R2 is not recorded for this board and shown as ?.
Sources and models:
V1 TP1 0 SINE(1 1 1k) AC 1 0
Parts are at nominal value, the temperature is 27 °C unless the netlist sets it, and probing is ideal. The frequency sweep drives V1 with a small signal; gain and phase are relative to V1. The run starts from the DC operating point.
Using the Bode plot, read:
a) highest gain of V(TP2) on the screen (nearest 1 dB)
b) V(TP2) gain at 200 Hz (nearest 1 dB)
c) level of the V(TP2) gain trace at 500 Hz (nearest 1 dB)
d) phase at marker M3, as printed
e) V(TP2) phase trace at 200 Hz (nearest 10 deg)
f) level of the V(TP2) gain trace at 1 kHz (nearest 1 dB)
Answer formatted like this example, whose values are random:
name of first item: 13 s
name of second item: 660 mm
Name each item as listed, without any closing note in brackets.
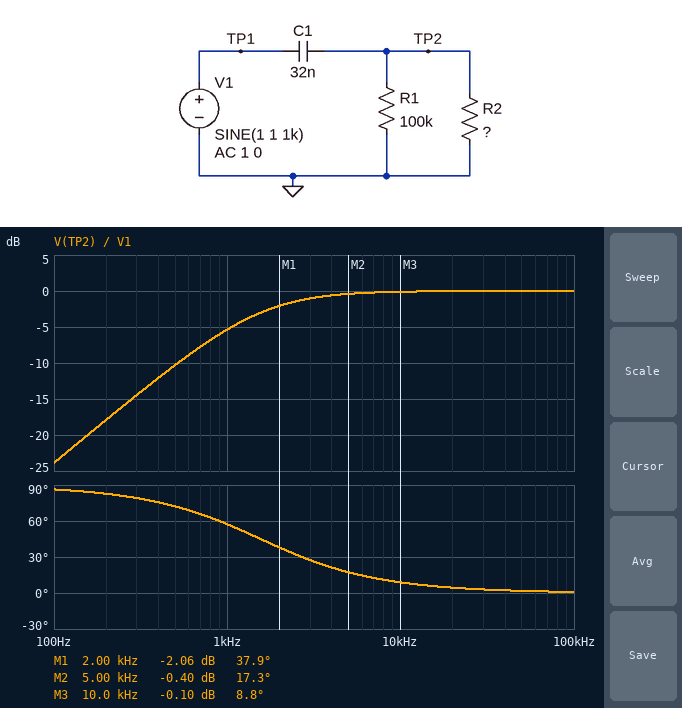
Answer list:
highest gain of V(TP2) on the screen: 0 dB
V(TP2) gain at 200 Hz: -18 dB
level of the V(TP2) gain trace at 500 Hz: -10 dB
phase at marker M3, as printed: 8.8 deg
V(TP2) phase trace at 200 Hz: 80 deg
level of the V(TP2) gain trace at 1 kHz: -5 dB
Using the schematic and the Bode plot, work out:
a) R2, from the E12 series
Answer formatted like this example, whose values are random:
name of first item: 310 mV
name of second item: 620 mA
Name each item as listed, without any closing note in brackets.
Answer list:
R2, from the E12 series: 3.3 kΩ
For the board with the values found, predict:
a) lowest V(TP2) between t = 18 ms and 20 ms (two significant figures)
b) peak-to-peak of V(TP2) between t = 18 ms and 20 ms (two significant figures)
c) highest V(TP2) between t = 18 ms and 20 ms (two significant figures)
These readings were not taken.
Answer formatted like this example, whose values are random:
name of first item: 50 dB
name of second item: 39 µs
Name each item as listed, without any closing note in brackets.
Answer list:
lowest V(TP2) between t = 18 ms and 20 ms: -540 mV
peak-to-peak of V(TP2) between t = 18 ms and 20 ms: 1.1 V
highest V(TP2) between t = 18 ms and 20 ms: 540 mV
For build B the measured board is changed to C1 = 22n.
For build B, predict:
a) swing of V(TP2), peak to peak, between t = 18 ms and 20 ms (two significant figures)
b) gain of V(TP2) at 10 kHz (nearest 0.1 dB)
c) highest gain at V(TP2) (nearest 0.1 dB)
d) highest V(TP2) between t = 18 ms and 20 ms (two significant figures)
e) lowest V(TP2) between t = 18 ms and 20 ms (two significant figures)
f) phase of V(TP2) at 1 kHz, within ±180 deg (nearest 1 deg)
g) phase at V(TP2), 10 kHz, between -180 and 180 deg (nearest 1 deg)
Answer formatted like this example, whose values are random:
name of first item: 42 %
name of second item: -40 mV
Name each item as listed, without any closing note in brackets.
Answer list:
swing of V(TP2), peak to peak, between t = 18 ms and 20 ms: 810 mV
gain of V(TP2) at 10 kHz: -0.2 dB
highest gain at V(TP2): 0 dB
highest V(TP2) between t = 18 ms and 20 ms: 400 mV
lowest V(TP2) between t = 18 ms and 20 ms: -400 mV
phase of V(TP2) at 1 kHz, within ±180 deg: 66 deg
phase at V(TP2), 10 kHz, between -180 and 180 deg: 13 deg
